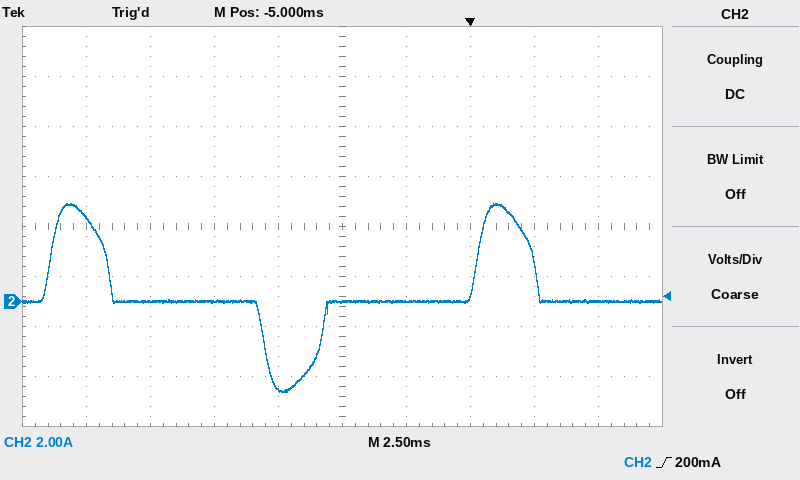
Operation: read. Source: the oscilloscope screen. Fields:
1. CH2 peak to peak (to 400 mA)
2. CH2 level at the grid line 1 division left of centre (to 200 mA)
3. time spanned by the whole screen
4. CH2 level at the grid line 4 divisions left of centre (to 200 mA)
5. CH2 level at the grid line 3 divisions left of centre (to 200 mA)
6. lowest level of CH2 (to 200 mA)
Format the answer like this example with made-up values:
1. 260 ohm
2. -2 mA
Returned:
1. 7.6 A
2. -3.4 A
3. 25 ms
4. 3.4 A
5. 0.0 A
6. -3.6 A
